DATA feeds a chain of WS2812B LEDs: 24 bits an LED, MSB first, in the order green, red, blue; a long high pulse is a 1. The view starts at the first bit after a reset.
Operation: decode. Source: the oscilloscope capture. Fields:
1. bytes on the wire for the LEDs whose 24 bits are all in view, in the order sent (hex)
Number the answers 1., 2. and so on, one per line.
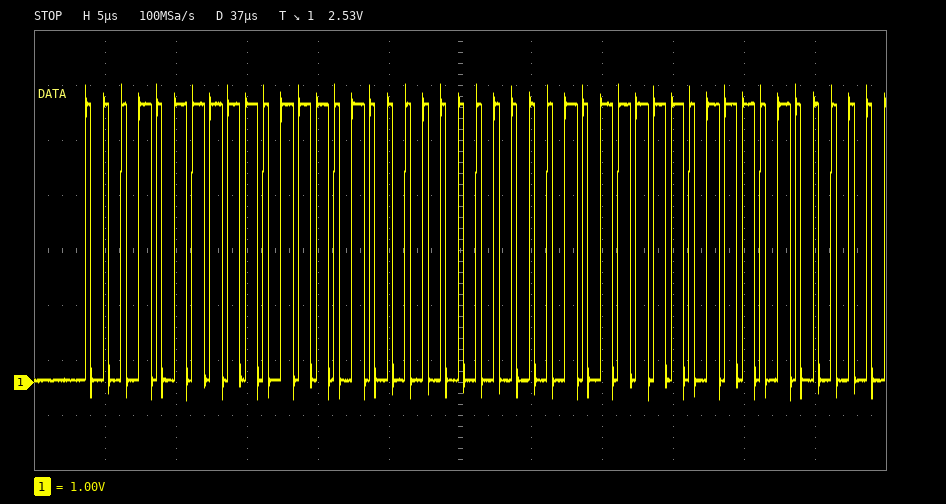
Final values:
1. 17 DD 00
